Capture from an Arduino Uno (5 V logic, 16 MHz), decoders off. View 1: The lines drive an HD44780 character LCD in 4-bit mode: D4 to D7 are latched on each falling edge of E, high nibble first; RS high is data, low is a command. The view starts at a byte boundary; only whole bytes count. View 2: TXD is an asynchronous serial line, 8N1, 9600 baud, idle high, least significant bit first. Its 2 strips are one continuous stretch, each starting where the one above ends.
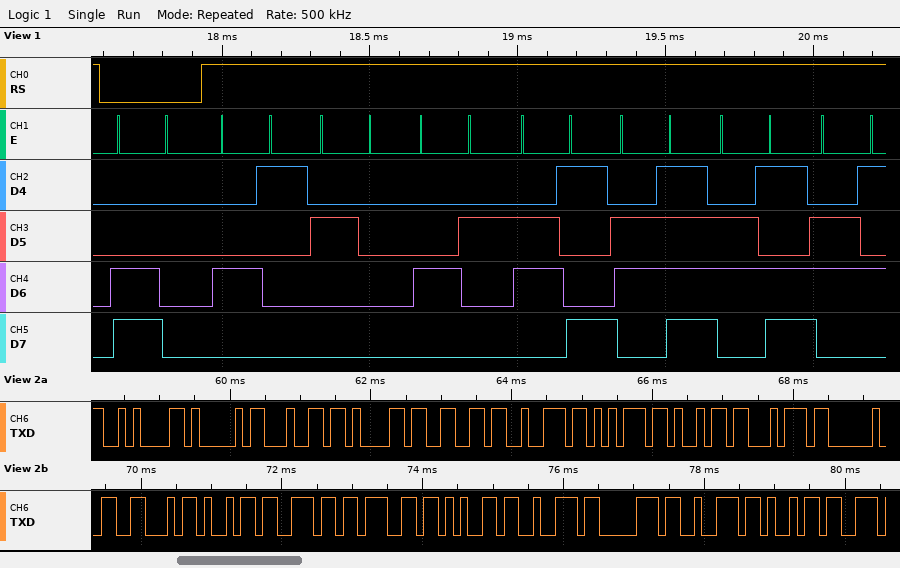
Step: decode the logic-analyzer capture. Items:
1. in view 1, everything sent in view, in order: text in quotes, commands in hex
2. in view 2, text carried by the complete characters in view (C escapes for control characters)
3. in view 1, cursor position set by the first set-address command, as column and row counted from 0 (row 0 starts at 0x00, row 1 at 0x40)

0xC0 "A Biome"
"\nAdafruit Fingerpri"
column 0, row 1
